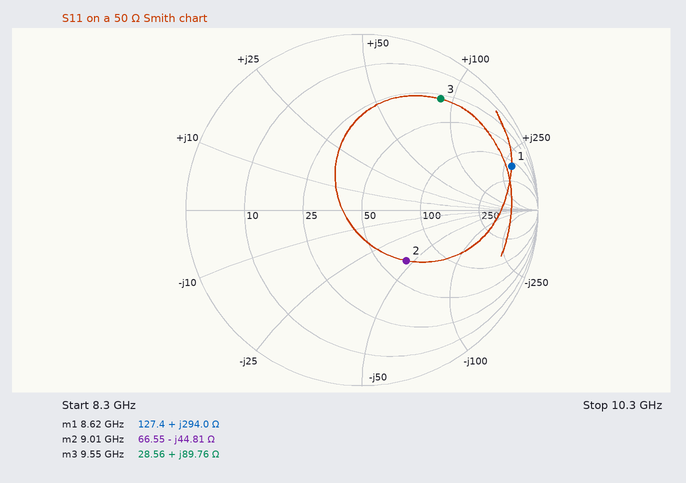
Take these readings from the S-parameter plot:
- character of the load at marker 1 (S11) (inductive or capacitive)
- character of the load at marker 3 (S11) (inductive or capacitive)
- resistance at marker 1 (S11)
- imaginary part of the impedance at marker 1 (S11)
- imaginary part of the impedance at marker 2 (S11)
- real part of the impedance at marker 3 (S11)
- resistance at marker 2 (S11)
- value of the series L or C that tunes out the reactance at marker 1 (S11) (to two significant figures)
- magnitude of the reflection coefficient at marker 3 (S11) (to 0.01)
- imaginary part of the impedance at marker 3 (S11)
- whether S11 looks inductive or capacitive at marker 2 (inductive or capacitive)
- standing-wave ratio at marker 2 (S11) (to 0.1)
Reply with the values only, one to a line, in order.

inductive
inductive
127.4 Ω
+294.0 Ω
-44.81 Ω
28.56 Ω
66.55 Ω
63 fF
0.77
+89.76 Ω
capacitive
2.2
